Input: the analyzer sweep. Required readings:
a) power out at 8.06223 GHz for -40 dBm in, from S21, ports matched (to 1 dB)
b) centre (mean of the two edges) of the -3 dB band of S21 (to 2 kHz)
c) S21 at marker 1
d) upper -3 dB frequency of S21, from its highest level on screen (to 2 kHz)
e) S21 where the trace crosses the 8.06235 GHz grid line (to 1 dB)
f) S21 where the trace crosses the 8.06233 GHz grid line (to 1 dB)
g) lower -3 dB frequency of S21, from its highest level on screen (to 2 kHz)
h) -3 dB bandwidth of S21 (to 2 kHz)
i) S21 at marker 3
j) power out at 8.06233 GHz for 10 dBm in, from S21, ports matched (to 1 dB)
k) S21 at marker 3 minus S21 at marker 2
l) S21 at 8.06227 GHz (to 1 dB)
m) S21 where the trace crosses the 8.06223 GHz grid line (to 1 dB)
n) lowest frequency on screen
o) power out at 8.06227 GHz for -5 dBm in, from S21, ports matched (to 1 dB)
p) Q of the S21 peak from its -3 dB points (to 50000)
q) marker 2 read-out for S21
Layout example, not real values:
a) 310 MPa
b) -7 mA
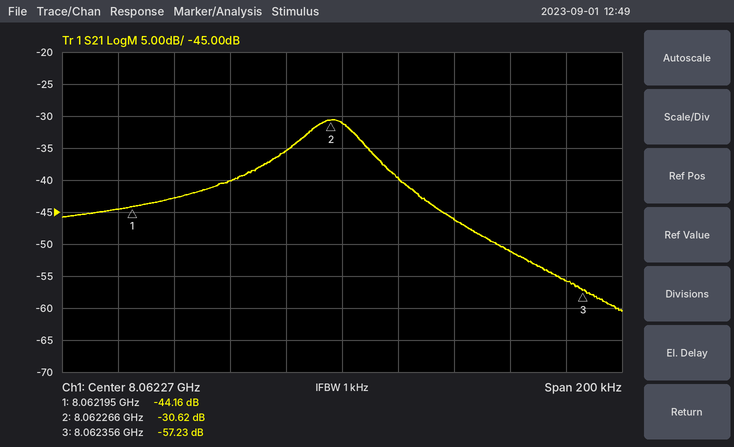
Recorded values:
a) -80 dBm
b) 8.062266 GHz
c) -44.16 dB
d) 8.062276 GHz
e) -56 dB
f) -51 dB
g) 8.062256 GHz
h) 20 kHz
i) -57.23 dB
j) -41 dBm
k) -26.61 dB
l) -31 dB
m) -40 dB
n) 8.06217 GHz
o) -36 dBm
p) 400000
q) -30.62 dB
